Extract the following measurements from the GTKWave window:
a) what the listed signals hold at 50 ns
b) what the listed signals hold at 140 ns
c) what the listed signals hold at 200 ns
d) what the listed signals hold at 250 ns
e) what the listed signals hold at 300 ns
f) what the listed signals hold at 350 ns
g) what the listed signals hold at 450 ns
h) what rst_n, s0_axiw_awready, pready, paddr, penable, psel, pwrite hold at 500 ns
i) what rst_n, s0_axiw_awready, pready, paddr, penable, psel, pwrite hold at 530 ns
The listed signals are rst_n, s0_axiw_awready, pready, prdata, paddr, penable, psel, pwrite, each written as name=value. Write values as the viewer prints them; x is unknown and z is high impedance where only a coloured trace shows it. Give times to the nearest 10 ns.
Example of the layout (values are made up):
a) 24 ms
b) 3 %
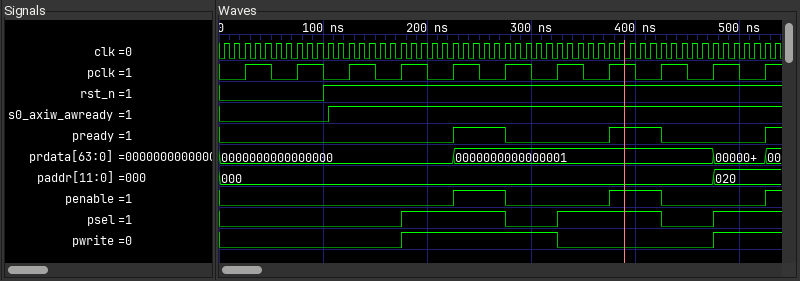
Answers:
a) rst_n=0, s0_axiw_awready=0, pready=0, prdata=0000000000000000, paddr=000, penable=0, psel=0, pwrite=0
b) rst_n=1, s0_axiw_awready=1, pready=0, prdata=0000000000000000, paddr=000, penable=0, psel=0, pwrite=0
c) rst_n=1, s0_axiw_awready=1, pready=0, prdata=0000000000000000, paddr=000, penable=0, psel=1, pwrite=1
d) rst_n=1, s0_axiw_awready=1, pready=1, prdata=0000000000000001, paddr=000, penable=1, psel=1, pwrite=1
e) rst_n=1, s0_axiw_awready=1, pready=0, prdata=0000000000000001, paddr=000, penable=0, psel=0, pwrite=1
f) rst_n=1, s0_axiw_awready=1, pready=0, prdata=0000000000000001, paddr=000, penable=0, psel=1, pwrite=0
g) rst_n=1, s0_axiw_awready=1, pready=0, prdata=0000000000000001, paddr=000, penable=0, psel=0, pwrite=0
h) rst_n=1, s0_axiw_awready=1, pready=0, paddr=020, penable=0, psel=1, pwrite=1
i) rst_n=1, s0_axiw_awready=1, pready=1, paddr=020, penable=1, psel=1, pwrite=1
